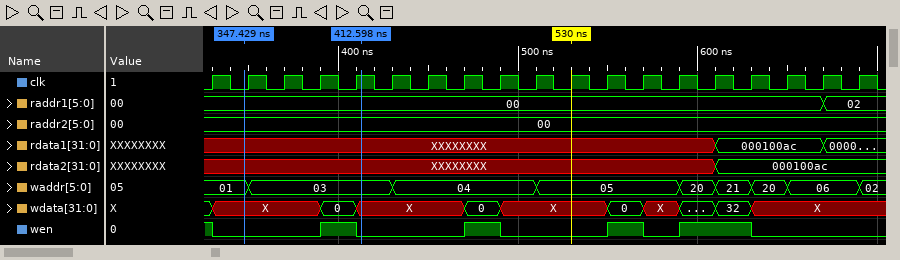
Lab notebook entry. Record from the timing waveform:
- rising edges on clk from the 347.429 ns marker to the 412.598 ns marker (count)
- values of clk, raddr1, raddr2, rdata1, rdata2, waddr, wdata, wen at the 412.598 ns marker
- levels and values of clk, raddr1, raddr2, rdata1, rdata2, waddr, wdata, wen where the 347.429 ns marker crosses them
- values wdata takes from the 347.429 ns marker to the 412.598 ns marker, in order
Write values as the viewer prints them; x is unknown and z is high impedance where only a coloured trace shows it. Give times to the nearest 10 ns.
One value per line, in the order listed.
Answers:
4
clk=1, raddr1=00, raddr2=00, rdata1=XXXXXXXX, rdata2=XXXXXXXX, waddr=03, wdata=X, wen=0
clk=0, raddr1=00, raddr2=00, rdata1=XXXXXXXX, rdata2=XXXXXXXX, waddr=01, wdata=X, wen=0
X, 0, X
